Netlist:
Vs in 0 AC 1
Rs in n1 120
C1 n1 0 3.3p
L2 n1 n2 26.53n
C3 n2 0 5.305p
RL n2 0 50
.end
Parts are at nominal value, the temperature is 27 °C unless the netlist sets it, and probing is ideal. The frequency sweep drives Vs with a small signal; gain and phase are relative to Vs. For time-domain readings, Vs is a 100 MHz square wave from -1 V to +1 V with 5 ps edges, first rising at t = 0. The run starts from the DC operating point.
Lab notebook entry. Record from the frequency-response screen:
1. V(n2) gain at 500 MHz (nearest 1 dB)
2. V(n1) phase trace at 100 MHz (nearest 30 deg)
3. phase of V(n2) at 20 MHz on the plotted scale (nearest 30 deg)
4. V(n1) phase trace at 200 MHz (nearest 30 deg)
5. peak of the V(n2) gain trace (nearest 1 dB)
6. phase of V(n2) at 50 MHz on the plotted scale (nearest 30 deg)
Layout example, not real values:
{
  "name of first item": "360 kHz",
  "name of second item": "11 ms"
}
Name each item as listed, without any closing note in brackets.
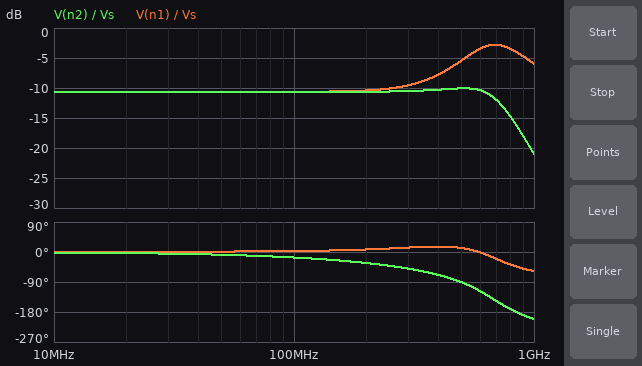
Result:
{
  "V(n2) gain at 500 MHz": "-10 dB",
  "V(n1) phase trace at 100 MHz": "0 deg",
  "phase of V(n2) at 20 MHz on the plotted scale": "0 deg",
  "V(n1) phase trace at 200 MHz": "0 deg",
  "peak of the V(n2) gain trace": "-10 dB",
  "phase of V(n2) at 50 MHz on the plotted scale": "0 deg"
}
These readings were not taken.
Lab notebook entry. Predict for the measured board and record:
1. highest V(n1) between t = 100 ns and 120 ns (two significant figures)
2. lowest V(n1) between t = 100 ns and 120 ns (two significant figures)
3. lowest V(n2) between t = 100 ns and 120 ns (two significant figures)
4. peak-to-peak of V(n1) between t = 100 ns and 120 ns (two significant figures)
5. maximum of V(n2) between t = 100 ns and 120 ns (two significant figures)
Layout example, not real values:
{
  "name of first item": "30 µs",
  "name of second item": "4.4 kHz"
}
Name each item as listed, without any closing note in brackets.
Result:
{
  "highest V(n1) between t = 100 ns and 120 ns": "650 mV",
  "lowest V(n1) between t = 100 ns and 120 ns": "-650 mV",
  "lowest V(n2) between t = 100 ns and 120 ns": "-370 mV",
  "peak-to-peak of V(n1) between t = 100 ns and 120 ns": "1.3 V",
  "maximum of V(n2) between t = 100 ns and 120 ns": "370 mV"
}
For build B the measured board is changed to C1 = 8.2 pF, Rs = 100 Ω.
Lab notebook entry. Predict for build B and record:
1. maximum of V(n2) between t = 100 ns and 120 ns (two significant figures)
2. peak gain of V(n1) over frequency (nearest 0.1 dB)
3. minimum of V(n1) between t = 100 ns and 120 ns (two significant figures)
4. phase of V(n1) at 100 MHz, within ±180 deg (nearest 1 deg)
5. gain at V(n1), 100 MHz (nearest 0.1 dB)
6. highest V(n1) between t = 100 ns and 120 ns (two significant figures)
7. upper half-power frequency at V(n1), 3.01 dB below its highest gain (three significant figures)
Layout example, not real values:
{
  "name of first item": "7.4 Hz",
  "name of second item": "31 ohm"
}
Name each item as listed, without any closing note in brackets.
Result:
{
  "maximum of V(n2) between t = 100 ns and 120 ns": "410 mV",
  "peak gain of V(n1) over frequency": "-6.3 dB",
  "minimum of V(n1) between t = 100 ns and 120 ns": "-480 mV",
  "phase of V(n1) at 100 MHz, within ±180 deg": "-3 deg",
  "gain at V(n1), 100 MHz": "-9.5 dB",
  "highest V(n1) between t = 100 ns and 120 ns": "480 mV",
  "upper half-power frequency at V(n1), 3.01 dB below its highest gain": "712 MHz"
}
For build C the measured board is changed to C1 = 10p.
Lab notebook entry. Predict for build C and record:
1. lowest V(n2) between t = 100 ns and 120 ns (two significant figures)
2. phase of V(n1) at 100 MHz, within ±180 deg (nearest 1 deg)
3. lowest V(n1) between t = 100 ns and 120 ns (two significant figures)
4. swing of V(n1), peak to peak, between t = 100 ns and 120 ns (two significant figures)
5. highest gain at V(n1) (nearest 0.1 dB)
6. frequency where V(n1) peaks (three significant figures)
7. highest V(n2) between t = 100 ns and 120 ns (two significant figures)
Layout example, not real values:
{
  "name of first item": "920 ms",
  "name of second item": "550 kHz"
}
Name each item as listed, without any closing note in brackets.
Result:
{
  "lowest V(n2) between t = 100 ns and 120 ns": "-350 mV",
  "phase of V(n1) at 100 MHz, within ±180 deg": "-6 deg",
  "lowest V(n1) between t = 100 ns and 120 ns": "-390 mV",
  "swing of V(n1), peak to peak, between t = 100 ns and 120 ns": "770 mV",
  "highest gain at V(n1)": "-8.5 dB",
  "frequency where V(n1) peaks": "431 MHz",
  "highest V(n2) between t = 100 ns and 120 ns": "350 mV"
}
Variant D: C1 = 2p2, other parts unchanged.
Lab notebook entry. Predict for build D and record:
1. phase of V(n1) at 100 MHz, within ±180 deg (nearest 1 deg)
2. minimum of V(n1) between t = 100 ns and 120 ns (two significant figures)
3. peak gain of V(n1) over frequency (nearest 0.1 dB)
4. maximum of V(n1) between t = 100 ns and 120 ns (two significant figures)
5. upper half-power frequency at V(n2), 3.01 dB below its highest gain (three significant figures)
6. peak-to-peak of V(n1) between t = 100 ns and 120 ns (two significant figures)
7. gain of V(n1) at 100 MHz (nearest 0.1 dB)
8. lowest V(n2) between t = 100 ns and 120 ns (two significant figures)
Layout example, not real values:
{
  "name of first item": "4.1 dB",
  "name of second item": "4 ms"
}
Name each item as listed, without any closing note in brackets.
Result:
{
  "phase of V(n1) at 100 MHz, within ±180 deg": "4 deg",
  "minimum of V(n1) between t = 100 ns and 120 ns": "-760 mV",
  "peak gain of V(n1) over frequency": "-1.6 dB",
  "maximum of V(n1) between t = 100 ns and 120 ns": "760 mV",
  "upper half-power frequency at V(n2), 3.01 dB below its highest gain": "833 MHz",
  "peak-to-peak of V(n1) between t = 100 ns and 120 ns": "1.5 V",
  "gain of V(n1) at 100 MHz": "-10.6 dB",
  "lowest V(n2) between t = 100 ns and 120 ns": "-350 mV"
}
